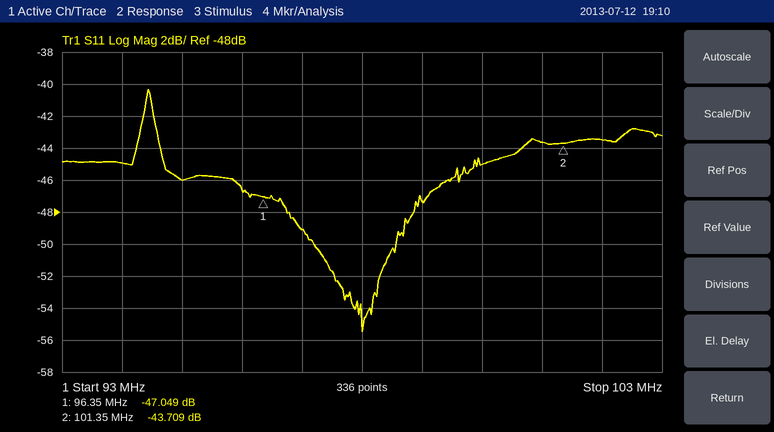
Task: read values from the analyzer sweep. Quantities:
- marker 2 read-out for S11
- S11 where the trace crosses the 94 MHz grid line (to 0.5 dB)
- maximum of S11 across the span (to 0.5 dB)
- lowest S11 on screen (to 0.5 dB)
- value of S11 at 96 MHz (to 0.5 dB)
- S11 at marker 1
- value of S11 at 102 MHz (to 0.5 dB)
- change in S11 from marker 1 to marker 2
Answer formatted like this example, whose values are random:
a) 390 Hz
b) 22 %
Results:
a) -43.709 dB
b) -45.0 dB
c) -40.5 dB
d) -55.5 dB
e) -46.5 dB
f) -47.049 dB
g) -43.5 dB
h) 3.340 dB
